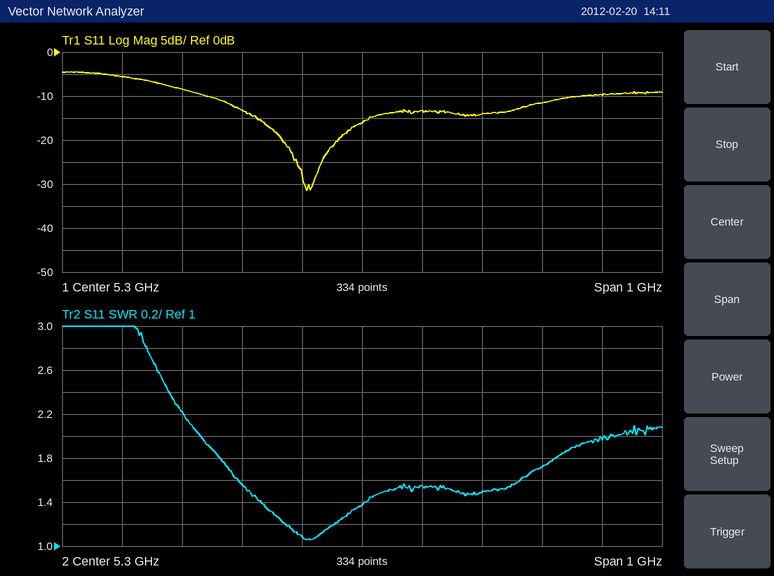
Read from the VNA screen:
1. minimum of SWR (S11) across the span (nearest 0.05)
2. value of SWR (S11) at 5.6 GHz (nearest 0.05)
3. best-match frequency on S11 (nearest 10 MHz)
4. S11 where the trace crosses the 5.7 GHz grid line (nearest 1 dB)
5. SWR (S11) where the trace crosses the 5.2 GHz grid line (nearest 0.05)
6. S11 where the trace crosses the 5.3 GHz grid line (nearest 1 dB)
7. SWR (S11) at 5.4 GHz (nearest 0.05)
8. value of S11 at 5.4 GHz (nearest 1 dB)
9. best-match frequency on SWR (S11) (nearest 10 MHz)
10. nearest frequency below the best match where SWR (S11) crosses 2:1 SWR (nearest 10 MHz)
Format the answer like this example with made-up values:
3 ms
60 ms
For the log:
1.05
1.70
5.21 GHz
-10 dB
1.10
-16 dB
1.55
-13 dB
5.21 GHz
5.03 GHz
